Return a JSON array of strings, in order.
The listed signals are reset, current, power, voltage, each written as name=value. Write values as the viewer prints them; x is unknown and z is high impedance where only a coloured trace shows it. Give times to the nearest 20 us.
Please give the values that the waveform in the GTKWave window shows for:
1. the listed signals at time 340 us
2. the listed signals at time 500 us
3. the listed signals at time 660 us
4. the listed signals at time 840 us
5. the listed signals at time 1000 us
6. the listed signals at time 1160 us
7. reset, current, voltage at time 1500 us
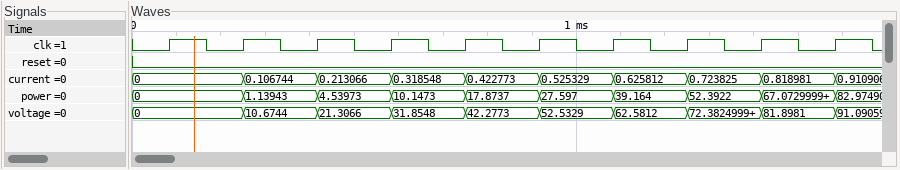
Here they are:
["reset=0, current=0.106744, power=1.13943, voltage=10.6744", "reset=0, current=0.213066, power=4.53973, voltage=21.3066", "reset=0, current=0.318548, power=10.1473, voltage=31.8548", "reset=0, current=0.422773, power=17.8737, voltage=42.2773", "reset=0, current=0.525329, power=27.597, voltage=52.5329", "reset=0, current=0.625812, power=39.164, voltage=62.5812", "reset=0, current=0.818981, voltage=81.8981"]
